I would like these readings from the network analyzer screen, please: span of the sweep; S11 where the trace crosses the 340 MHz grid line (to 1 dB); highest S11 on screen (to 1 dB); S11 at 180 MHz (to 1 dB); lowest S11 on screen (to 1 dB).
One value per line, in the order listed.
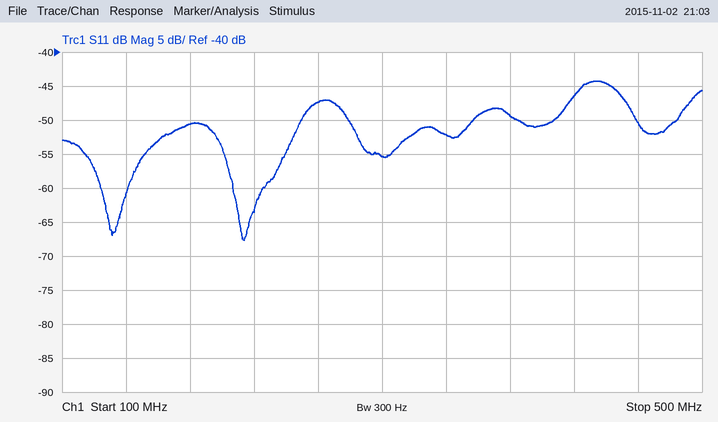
400 MHz
-52 dB
-44 dB
-51 dB
-68 dB
